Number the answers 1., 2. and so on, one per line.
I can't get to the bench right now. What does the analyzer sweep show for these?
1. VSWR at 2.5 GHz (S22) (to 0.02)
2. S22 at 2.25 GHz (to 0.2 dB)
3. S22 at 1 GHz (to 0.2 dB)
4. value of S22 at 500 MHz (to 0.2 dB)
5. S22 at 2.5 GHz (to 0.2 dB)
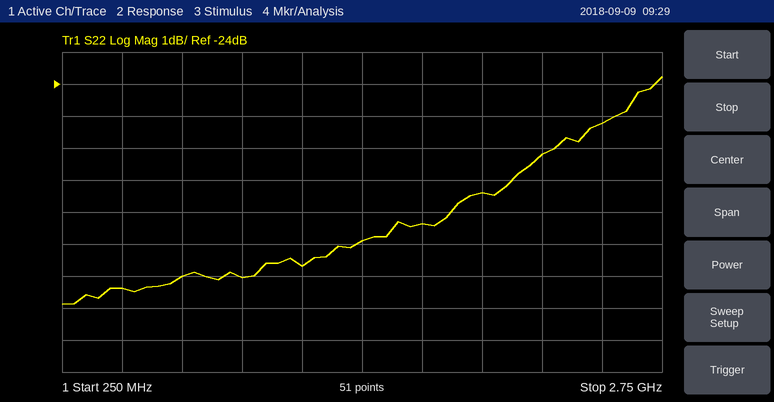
1. 1.12
2. -26.2 dB
3. -30.0 dB
4. -30.4 dB
5. -25.2 dB
